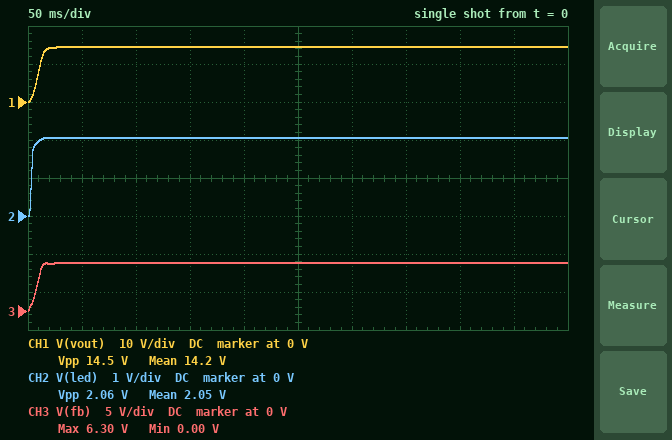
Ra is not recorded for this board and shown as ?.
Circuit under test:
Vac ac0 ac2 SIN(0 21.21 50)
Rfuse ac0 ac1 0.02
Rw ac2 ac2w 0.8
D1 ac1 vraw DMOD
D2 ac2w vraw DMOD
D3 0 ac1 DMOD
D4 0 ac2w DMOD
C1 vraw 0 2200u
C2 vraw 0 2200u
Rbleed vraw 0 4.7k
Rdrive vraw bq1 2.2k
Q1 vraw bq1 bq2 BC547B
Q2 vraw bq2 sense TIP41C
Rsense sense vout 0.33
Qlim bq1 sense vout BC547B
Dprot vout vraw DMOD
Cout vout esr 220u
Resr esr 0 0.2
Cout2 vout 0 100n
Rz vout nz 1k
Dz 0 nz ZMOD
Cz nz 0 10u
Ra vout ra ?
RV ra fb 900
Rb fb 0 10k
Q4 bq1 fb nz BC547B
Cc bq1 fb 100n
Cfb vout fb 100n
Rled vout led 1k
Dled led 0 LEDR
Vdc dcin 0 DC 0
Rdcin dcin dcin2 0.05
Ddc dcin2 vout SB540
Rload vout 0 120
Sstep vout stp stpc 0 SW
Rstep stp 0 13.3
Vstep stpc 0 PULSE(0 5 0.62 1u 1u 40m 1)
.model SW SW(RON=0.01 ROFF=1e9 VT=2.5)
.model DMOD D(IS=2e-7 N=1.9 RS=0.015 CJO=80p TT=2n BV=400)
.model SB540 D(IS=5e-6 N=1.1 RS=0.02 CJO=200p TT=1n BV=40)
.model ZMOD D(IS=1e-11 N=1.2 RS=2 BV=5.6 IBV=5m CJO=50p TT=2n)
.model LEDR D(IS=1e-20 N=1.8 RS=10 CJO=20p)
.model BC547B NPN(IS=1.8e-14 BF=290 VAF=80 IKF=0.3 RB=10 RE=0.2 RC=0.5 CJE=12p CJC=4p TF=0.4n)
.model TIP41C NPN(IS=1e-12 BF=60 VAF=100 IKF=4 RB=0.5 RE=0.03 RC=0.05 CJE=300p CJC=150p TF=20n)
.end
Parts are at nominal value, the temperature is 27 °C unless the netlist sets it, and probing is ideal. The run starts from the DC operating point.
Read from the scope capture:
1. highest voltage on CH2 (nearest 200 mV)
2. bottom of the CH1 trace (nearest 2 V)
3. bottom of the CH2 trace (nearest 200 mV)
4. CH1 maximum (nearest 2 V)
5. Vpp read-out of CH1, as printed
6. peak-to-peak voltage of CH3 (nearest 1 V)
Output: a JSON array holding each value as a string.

["2.0 V", "0 V", "0 V", "14 V", "14.5 V", "6 V"]
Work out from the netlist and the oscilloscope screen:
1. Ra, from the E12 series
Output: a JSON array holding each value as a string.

["12 kΩ"]
